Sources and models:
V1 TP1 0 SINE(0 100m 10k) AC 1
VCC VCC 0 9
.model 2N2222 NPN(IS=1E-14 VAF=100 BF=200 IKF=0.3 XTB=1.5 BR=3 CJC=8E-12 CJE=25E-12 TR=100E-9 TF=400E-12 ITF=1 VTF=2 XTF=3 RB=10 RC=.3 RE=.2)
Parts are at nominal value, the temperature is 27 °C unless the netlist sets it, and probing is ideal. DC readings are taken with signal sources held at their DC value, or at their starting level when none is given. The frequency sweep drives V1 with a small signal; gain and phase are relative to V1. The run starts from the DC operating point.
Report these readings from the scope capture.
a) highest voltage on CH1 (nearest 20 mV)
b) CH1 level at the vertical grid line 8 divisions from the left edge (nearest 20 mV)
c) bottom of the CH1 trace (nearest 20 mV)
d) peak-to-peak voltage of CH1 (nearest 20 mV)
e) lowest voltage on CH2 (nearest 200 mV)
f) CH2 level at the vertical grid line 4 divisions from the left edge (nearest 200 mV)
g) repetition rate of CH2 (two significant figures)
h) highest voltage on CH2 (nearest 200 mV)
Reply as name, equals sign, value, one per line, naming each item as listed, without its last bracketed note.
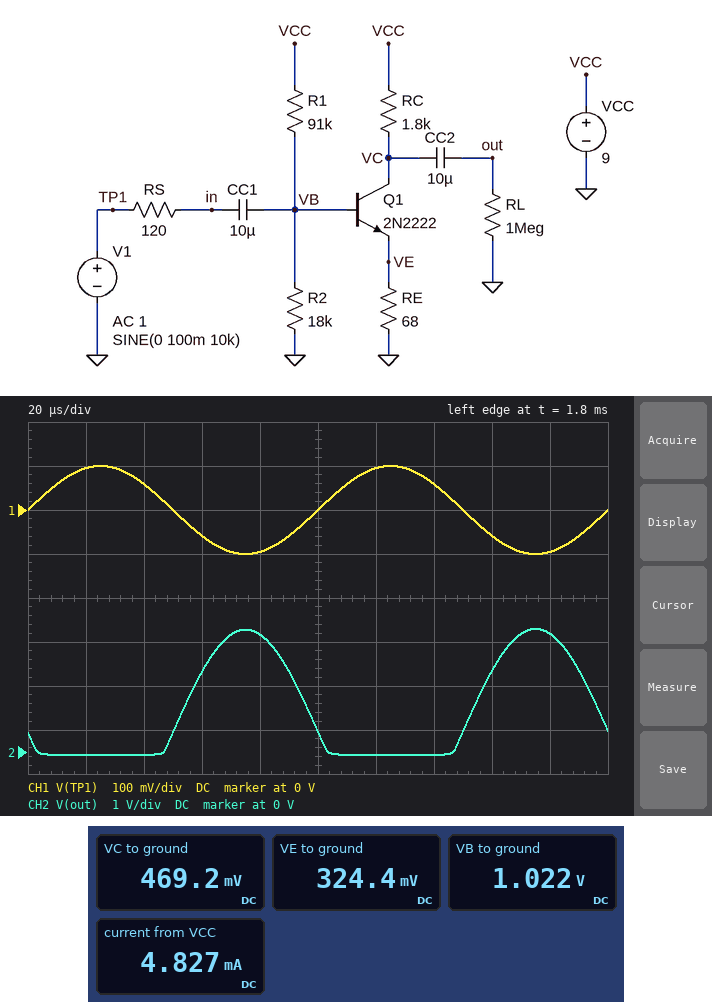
highest voltage on CH1 = 100 mV
CH1 level at the vertical grid line 8 divisions from the left edge = -60 mV
bottom of the CH1 trace = -100 mV
peak-to-peak voltage of CH1 = 200 mV
lowest voltage on CH2 = 0 V
CH2 level at the vertical grid line 4 divisions from the left edge = 2.6 V
repetition rate of CH2 = 10 kHz
highest voltage on CH2 = 2.8 V
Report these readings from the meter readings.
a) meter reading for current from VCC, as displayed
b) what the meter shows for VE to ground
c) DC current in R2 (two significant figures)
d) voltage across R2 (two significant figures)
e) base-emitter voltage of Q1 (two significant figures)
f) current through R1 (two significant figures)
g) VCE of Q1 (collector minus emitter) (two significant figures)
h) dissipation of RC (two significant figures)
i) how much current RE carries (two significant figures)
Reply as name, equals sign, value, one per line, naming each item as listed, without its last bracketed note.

meter reading for current from VCC, as displayed = 4.827 mA
what the meter shows for VE to ground = 324.4 mV
DC current in R2 = 57 µA
voltage across R2 = 1.0 V
base-emitter voltage of Q1 = 700 mV
current through R1 = 88 µA
VCE of Q1 (collector minus emitter) = 140 mV
dissipation of RC = 40 mW
how much current RE carries = 4.8 mA
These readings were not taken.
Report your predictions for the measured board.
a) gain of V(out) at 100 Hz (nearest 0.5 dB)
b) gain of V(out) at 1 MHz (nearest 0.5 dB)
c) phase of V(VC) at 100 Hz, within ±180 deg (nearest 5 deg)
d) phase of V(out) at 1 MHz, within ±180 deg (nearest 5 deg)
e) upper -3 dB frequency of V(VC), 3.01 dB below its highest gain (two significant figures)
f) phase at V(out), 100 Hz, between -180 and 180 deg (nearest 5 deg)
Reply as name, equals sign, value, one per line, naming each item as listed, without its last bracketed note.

gain of V(out) at 100 Hz = 19.0 dB
gain of V(out) at 1 MHz = 16.0 dB
phase of V(VC) at 100 Hz, within ±180 deg = -155 deg
phase of V(out) at 1 MHz, within ±180 deg = 130 deg
upper -3 dB frequency of V(VC), 3.01 dB below its highest gain = 860 kHz
phase at V(out), 100 Hz, between -180 and 180 deg = -155 deg
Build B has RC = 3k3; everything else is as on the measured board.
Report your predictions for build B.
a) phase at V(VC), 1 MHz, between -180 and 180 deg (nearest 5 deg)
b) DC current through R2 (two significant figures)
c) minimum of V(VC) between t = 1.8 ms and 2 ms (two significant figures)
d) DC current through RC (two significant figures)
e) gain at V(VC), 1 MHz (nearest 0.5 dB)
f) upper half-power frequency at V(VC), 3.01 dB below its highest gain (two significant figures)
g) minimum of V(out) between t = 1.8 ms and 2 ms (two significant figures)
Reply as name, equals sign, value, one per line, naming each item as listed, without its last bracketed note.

phase at V(VC), 1 MHz, between -180 and 180 deg = 110 deg
DC current through R2 = 48 µA
minimum of V(VC) between t = 1.8 ms and 2 ms = 240 mV
DC current through RC = 2.6 mA
gain at V(VC), 1 MHz = 4.5 dB
upper half-power frequency at V(VC), 3.01 dB below its highest gain = 650 kHz
minimum of V(out) between t = 1.8 ms and 2 ms = -34 mV
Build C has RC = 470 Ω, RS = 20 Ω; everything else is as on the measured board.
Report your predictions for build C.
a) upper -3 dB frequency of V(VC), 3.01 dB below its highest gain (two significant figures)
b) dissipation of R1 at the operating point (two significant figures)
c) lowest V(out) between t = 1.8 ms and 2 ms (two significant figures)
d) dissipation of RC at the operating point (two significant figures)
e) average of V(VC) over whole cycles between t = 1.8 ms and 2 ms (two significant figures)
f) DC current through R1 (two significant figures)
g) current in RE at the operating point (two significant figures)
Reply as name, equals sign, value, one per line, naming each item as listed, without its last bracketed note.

upper -3 dB frequency of V(VC), 3.01 dB below its highest gain = 53 MHz
dissipation of R1 at the operating point = 690 µW
lowest V(out) between t = 1.8 ms and 2 ms = -640 mV
dissipation of RC at the operating point = 15 mW
average of V(VC) over whole cycles between t = 1.8 ms and 2 ms = 6.4 V
DC current through R1 = 87 µA
current in RE at the operating point = 5.6 mA
